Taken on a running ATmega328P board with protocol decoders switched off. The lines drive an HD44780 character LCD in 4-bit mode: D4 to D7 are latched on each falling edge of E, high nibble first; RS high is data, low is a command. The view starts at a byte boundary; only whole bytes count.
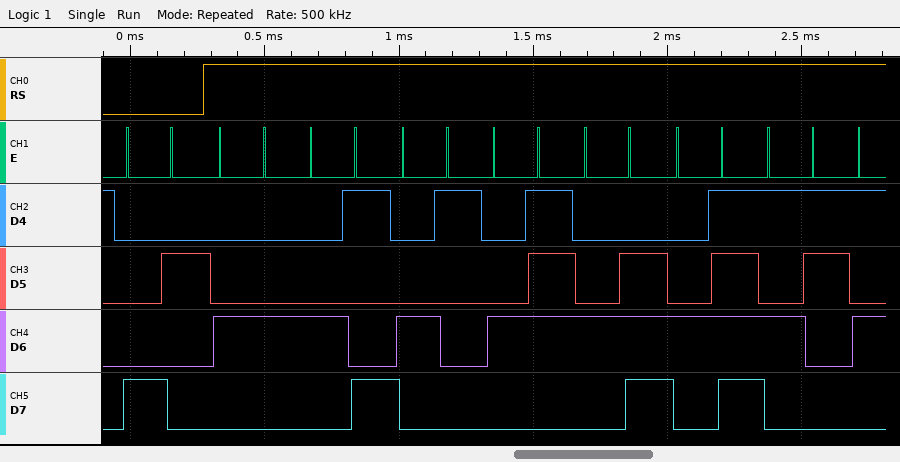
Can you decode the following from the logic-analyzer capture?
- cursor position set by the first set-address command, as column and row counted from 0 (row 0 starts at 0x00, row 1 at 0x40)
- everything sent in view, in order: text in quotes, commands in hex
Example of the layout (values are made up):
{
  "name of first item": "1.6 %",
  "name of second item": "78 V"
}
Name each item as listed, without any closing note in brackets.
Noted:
{
  "cursor position set by the first set-address command, as column and row counted from 0": "column 2, row 0",
  "everything sent in view, in order: text in quotes, commands in hex": "0x82 \"DIAGNOS\""
}
